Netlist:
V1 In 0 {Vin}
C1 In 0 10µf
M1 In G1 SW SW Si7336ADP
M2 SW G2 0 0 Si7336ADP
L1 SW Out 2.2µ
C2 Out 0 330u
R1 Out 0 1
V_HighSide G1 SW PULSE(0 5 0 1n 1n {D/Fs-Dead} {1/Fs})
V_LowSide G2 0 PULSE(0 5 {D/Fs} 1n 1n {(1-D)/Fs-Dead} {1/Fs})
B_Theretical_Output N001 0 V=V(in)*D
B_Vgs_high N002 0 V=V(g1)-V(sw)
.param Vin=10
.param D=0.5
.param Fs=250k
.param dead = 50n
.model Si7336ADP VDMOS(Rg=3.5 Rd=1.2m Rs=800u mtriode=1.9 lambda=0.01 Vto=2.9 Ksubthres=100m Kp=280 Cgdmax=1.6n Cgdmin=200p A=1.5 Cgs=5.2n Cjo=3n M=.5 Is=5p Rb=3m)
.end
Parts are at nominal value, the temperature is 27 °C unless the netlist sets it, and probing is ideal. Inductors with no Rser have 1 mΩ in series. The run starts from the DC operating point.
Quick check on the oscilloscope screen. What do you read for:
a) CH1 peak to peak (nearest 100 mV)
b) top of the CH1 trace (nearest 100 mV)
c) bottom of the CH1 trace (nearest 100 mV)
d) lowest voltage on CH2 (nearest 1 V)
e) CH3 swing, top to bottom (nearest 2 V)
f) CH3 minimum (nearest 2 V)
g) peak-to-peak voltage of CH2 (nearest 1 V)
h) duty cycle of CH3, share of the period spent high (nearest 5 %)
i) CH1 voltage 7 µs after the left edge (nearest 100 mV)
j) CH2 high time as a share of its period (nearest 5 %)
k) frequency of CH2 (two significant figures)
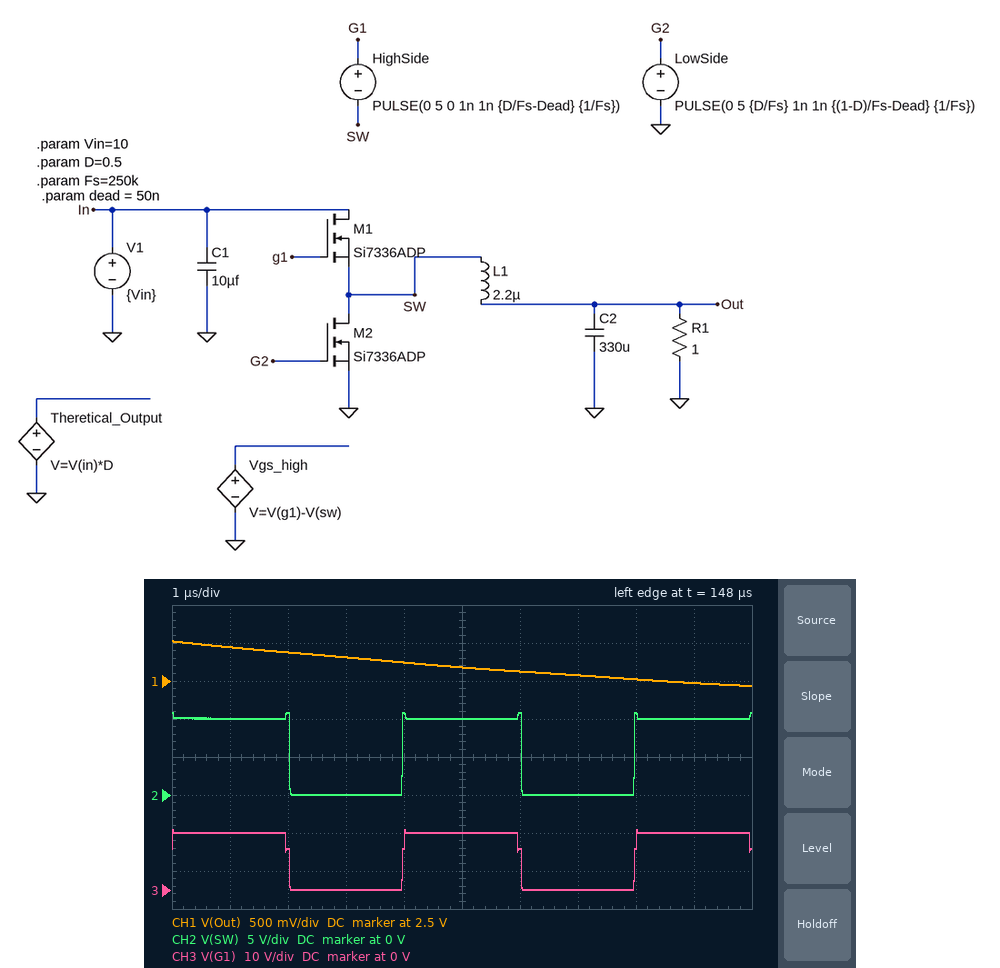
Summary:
600 mV
3.0 V
2.4 V
0 V
16 V
0 V
11 V
50 %
2.6 V
50 %
250 kHz
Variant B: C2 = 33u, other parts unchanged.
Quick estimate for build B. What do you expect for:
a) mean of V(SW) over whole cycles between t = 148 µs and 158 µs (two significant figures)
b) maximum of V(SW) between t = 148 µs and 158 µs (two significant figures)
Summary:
4.8 V
10 V
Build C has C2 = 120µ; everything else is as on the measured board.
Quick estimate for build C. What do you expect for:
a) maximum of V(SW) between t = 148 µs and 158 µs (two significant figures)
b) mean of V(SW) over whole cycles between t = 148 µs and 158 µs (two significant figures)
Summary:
10 V
4.8 V
